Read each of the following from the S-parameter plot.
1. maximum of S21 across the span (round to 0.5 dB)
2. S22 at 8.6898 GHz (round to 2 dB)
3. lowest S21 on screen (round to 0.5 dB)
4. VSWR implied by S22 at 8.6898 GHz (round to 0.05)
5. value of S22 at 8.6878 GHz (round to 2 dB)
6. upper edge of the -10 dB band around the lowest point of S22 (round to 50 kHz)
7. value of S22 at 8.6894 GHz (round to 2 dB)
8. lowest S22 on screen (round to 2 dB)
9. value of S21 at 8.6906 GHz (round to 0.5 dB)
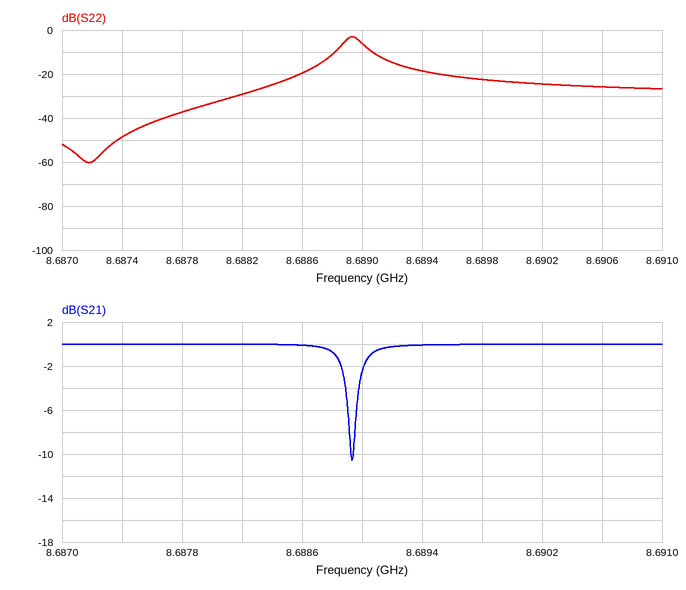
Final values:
0.0 dB
-22 dB
-10.5 dB
1.15
-38 dB
8.68880 GHz
-18 dB
-60 dB
0.0 dB
